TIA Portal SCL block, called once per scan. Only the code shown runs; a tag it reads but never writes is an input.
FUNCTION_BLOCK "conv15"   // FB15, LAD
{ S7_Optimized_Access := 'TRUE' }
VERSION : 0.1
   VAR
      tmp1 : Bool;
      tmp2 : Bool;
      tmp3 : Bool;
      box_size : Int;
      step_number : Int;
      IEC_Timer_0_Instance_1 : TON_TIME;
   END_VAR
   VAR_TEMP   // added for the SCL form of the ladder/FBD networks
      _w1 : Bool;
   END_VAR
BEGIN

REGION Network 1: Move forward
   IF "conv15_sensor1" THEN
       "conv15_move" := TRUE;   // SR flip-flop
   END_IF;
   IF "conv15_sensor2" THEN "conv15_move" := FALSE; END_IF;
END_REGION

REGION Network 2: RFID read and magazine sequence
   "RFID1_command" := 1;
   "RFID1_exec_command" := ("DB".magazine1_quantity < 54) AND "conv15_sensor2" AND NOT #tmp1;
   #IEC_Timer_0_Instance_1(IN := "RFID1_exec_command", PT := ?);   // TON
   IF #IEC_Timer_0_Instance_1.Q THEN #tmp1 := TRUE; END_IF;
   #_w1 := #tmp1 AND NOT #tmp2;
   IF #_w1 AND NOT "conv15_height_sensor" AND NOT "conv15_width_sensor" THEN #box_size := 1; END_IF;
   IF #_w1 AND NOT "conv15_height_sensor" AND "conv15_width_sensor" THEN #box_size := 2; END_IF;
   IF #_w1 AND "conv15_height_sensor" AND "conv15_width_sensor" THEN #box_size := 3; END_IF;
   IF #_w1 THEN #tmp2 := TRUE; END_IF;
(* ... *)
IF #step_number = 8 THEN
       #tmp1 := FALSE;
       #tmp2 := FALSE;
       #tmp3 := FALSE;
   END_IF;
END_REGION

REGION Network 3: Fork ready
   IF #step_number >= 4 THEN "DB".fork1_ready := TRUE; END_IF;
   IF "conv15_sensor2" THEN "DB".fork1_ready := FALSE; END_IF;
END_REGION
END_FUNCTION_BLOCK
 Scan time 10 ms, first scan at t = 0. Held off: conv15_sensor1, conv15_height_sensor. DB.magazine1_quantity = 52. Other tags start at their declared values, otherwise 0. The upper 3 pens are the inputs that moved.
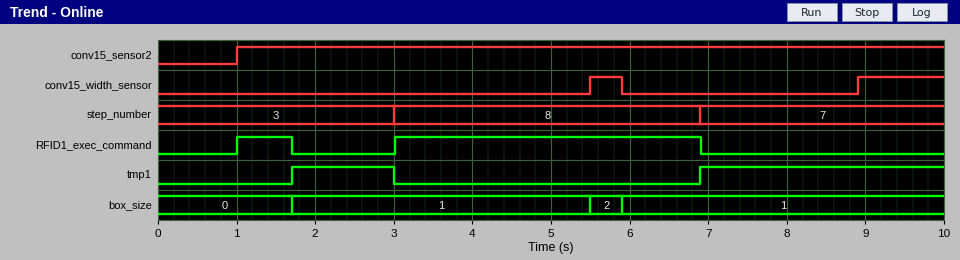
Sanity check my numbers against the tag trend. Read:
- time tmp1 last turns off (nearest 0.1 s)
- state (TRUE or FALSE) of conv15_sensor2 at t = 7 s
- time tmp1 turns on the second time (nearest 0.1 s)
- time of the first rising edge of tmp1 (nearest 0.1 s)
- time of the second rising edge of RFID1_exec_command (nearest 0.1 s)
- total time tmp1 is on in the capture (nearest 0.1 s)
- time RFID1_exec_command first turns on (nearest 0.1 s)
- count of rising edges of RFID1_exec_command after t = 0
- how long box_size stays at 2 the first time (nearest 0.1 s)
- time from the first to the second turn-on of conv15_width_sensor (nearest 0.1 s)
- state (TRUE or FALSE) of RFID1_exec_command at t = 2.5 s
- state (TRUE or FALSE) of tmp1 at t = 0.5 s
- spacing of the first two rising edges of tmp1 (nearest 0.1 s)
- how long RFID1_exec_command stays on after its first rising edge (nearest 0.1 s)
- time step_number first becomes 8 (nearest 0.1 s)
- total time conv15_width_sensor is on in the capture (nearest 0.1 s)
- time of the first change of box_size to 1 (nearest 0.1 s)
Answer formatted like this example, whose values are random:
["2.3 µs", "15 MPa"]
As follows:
["3.0 s", "TRUE", "6.9 s", "1.7 s", "3.0 s", "4.4 s", "1.0 s", "2", "0.4 s", "3.4 s", "FALSE", "FALSE", "5.2 s", "0.7 s", "3.0 s", "1.5 s", "1.7 s"]
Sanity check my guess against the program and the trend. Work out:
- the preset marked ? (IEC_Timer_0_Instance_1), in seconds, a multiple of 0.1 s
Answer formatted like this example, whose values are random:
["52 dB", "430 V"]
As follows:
["0.7 s"]
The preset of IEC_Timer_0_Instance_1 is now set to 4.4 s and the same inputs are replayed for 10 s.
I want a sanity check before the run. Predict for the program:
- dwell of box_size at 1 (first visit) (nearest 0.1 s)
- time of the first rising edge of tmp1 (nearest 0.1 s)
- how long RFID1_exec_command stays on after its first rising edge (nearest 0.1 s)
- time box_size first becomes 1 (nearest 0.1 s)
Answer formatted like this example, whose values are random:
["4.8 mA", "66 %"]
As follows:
["0.1 s", "6.9 s", "5.9 s", "5.4 s"]
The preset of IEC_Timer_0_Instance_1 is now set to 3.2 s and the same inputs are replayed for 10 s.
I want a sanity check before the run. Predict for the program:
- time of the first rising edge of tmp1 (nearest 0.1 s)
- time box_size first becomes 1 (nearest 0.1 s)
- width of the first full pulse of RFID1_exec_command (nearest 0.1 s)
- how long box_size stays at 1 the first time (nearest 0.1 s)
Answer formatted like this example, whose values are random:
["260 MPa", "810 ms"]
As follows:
["6.9 s", "4.2 s", "5.9 s", "1.3 s"]
